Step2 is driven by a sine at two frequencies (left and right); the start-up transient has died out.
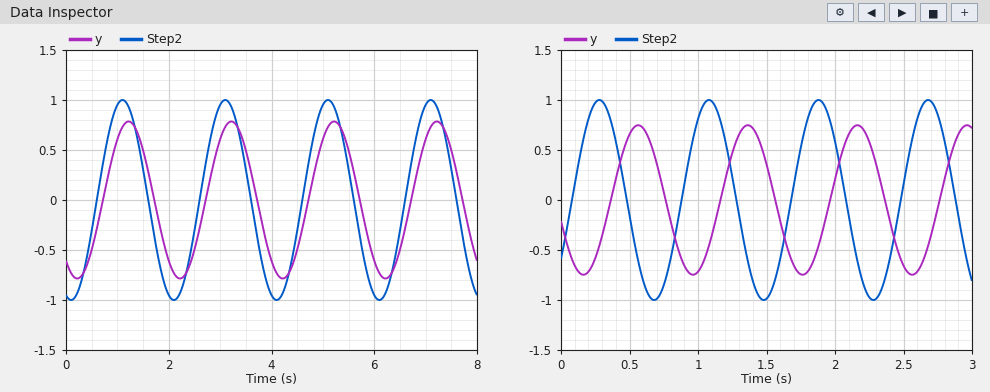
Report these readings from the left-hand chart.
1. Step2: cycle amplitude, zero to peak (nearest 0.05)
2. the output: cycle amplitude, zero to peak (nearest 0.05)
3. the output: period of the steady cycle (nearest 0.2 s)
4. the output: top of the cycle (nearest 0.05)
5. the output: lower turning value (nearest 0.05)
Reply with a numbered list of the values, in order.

1. 1.00
2. 0.80
3. 2.0 s
4. 0.80
5. -0.80
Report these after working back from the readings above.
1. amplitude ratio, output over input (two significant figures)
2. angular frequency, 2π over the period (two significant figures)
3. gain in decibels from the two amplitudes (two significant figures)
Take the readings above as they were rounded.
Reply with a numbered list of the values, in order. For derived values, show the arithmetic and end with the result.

1. 0.8 / 1 = 0.80
2. 2π / 2 = 3.1 rad/s
3. 20 log10(0.8 / 1) = -1.9 dB
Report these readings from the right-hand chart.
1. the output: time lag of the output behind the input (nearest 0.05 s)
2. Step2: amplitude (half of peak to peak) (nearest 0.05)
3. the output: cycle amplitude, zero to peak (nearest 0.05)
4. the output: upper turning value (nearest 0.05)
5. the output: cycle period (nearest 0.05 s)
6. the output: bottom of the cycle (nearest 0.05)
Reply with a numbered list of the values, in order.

1. 0.30 s
2. 1.00
3. 0.75
4. 0.75
5. 0.80 s
6. -0.75
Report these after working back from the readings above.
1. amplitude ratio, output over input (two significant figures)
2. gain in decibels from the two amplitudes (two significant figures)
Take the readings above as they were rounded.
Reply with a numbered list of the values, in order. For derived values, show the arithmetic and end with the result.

1. 0.75 / 1 = 0.75
2. 20 log10(0.75 / 1) = -2.5 dB
